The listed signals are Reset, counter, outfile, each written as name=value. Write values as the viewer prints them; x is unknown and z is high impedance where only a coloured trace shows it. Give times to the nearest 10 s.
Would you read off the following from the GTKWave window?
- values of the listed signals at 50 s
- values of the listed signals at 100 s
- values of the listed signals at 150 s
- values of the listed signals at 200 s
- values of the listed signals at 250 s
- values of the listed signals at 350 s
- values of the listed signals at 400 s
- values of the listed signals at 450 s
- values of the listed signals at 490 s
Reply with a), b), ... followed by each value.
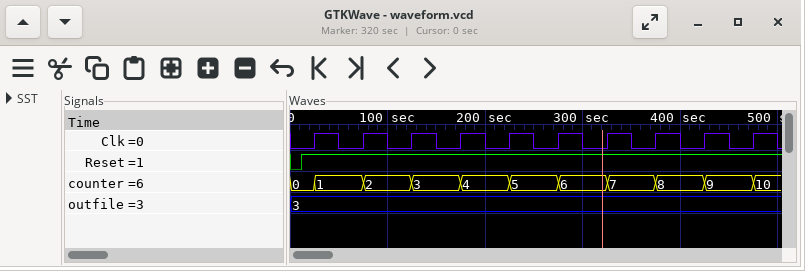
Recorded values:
a) Reset=1, counter=1, outfile=3
b) Reset=1, counter=2, outfile=3
c) Reset=1, counter=3, outfile=3
d) Reset=1, counter=4, outfile=3
e) Reset=1, counter=5, outfile=3
f) Reset=1, counter=7, outfile=3
g) Reset=1, counter=8, outfile=3
h) Reset=1, counter=9, outfile=3
i) Reset=1, counter=10, outfile=3
